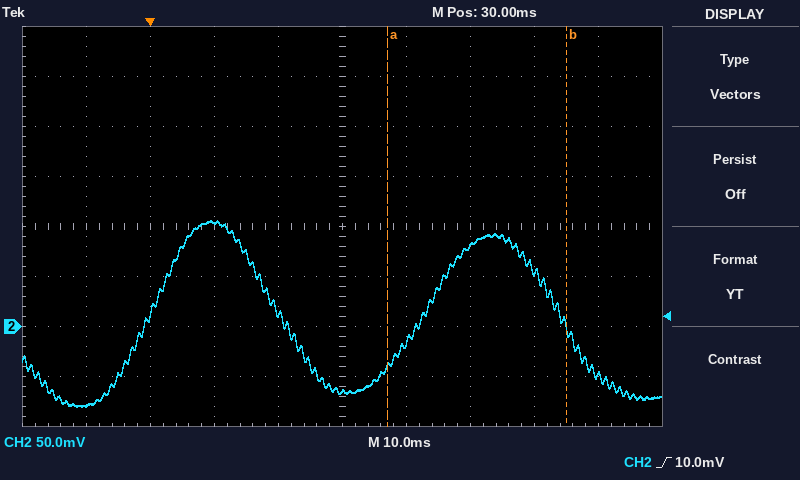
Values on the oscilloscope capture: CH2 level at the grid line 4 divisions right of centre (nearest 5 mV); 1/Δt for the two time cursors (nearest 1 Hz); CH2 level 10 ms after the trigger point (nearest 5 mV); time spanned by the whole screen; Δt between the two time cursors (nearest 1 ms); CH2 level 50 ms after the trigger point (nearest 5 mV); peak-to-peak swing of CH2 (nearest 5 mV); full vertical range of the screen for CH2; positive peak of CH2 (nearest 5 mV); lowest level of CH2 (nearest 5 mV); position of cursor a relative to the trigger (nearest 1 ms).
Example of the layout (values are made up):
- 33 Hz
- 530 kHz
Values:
- -50 mV
- 36 Hz
- 105 mV
- 100 ms
- 28 ms
- 80 mV
- 185 mV
- 400 mV
- 105 mV
- -80 mV
- +37 ms
